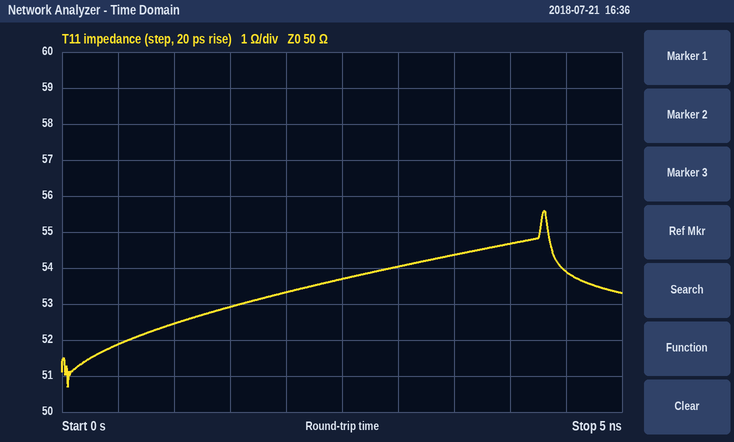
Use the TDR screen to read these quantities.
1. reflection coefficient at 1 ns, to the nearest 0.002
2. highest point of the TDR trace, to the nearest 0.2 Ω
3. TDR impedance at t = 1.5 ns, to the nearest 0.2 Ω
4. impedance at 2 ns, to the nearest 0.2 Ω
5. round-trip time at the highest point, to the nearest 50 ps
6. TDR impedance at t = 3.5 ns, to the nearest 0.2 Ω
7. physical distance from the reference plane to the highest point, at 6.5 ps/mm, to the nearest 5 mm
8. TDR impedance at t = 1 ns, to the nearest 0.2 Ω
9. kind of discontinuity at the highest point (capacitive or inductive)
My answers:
+0.024
55.6 Ω
53.0 Ω
53.4 Ω
4.30 ns
54.4 Ω
330 mm
52.4 Ω
inductive
